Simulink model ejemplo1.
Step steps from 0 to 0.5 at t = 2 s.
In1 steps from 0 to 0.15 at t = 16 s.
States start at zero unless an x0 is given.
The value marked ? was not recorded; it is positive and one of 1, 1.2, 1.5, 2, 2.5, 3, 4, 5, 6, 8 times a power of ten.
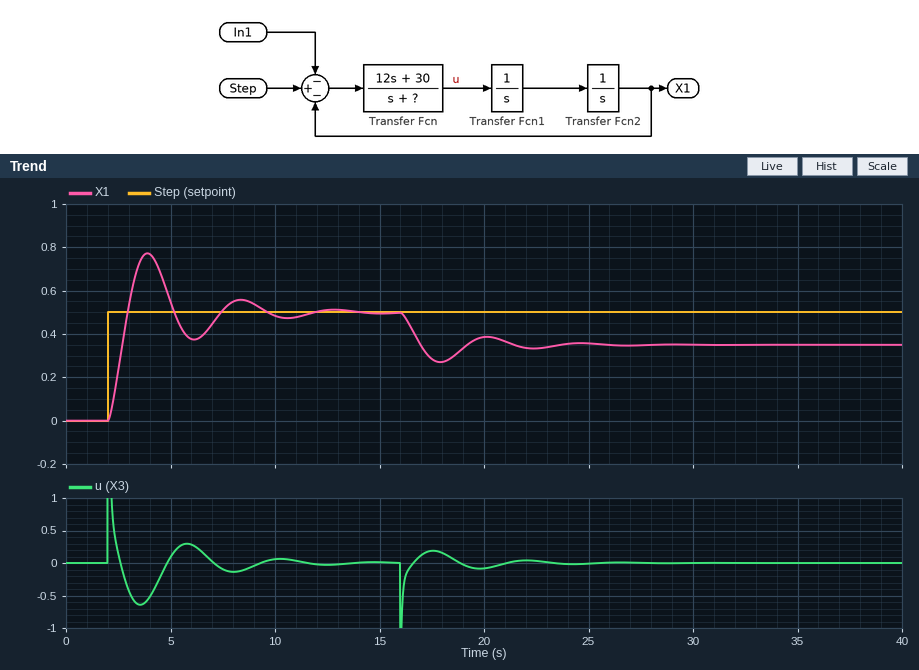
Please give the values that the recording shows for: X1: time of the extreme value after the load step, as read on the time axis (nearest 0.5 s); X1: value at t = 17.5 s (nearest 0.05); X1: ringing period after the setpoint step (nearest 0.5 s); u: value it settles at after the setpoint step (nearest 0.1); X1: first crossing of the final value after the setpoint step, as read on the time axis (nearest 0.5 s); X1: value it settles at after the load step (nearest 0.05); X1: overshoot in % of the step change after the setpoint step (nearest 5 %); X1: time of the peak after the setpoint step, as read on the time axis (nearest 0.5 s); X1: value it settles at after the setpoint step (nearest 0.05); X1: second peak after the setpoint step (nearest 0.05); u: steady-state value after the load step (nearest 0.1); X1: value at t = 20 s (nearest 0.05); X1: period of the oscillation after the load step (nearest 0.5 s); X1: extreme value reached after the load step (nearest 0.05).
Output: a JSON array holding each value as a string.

["18.0 s", "0.30", "4.5 s", "0.0", "3.0 s", "0.35", "55 %", "4.0 s", "0.50", "0.55", "0.0", "0.40", "4.5 s", "0.25"]
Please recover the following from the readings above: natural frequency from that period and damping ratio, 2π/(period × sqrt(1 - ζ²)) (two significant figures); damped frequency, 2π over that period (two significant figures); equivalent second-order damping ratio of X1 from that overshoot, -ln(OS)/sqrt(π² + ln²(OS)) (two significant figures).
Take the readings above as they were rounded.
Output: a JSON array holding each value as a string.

["1.4 rad/s", "1.4 rad/s", "0.19"]
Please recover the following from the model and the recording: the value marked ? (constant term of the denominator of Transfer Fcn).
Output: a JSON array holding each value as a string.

["15"]
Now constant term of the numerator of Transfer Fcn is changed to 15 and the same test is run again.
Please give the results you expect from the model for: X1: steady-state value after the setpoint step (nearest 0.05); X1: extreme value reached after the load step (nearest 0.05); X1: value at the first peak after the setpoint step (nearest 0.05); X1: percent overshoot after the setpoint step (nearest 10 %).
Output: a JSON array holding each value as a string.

["0.50", "0.30", "0.70", "40 %"]
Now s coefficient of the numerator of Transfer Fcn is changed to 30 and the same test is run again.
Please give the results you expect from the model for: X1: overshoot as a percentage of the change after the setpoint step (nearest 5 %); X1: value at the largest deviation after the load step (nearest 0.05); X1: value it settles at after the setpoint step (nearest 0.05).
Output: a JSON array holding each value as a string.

["25 %", "0.30", "0.50"]
